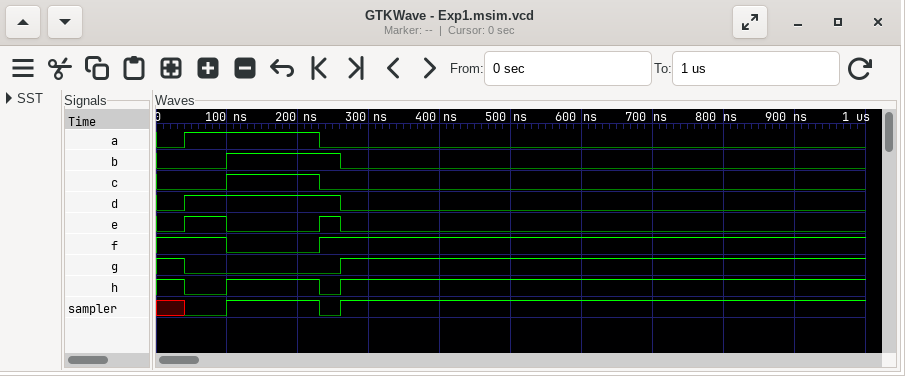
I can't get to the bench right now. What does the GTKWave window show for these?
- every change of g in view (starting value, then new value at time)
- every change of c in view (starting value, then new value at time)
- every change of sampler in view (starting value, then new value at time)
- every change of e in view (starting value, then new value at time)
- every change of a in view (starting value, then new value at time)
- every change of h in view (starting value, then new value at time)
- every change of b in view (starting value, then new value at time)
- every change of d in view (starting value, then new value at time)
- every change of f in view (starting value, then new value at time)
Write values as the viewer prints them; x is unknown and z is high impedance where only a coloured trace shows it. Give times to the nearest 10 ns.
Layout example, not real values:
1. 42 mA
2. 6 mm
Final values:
1. 1, 0 at 40 ns, 1 at 260 ns
2. 0, 1 at 100 ns, 0 at 230 ns
3. x, 0 at 40 ns, 1 at 100 ns, 0 at 230 ns, 1 at 260 ns
4. 0, 1 at 40 ns, 0 at 100 ns, 1 at 230 ns, 0 at 260 ns
5. 0, 1 at 40 ns, 0 at 230 ns
6. 1, 0 at 40 ns, 1 at 100 ns, 0 at 230 ns, 1 at 260 ns
7. 0, 1 at 100 ns, 0 at 260 ns
8. 0, 1 at 40 ns, 0 at 260 ns
9. 1, 0 at 100 ns, 1 at 230 ns
